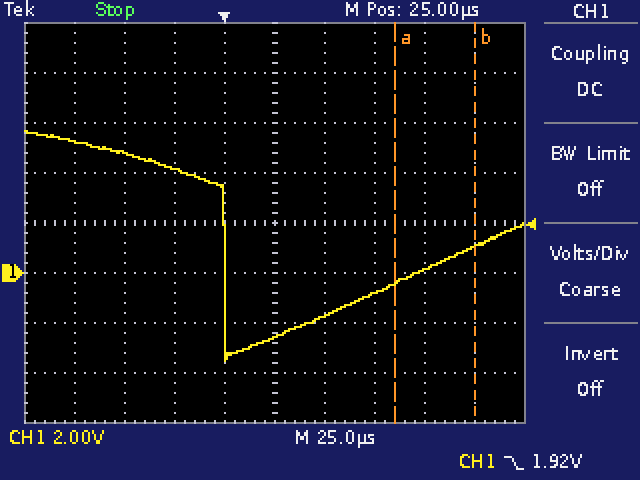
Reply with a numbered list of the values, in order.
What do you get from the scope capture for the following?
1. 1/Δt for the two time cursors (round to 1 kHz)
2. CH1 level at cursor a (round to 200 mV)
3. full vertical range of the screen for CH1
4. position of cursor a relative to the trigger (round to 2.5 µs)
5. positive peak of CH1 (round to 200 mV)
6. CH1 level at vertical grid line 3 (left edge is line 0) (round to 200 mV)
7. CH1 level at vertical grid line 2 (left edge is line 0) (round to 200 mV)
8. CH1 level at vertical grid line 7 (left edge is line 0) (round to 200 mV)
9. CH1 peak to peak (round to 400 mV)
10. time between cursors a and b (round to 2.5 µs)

1. 25 kHz
2. -400 mV
3. 16 V
4. +85.0 µs
5. 5.6 V
6. 4.2 V
7. 4.8 V
8. -800 mV
9. 9.2 V
10. 40.0 µs
